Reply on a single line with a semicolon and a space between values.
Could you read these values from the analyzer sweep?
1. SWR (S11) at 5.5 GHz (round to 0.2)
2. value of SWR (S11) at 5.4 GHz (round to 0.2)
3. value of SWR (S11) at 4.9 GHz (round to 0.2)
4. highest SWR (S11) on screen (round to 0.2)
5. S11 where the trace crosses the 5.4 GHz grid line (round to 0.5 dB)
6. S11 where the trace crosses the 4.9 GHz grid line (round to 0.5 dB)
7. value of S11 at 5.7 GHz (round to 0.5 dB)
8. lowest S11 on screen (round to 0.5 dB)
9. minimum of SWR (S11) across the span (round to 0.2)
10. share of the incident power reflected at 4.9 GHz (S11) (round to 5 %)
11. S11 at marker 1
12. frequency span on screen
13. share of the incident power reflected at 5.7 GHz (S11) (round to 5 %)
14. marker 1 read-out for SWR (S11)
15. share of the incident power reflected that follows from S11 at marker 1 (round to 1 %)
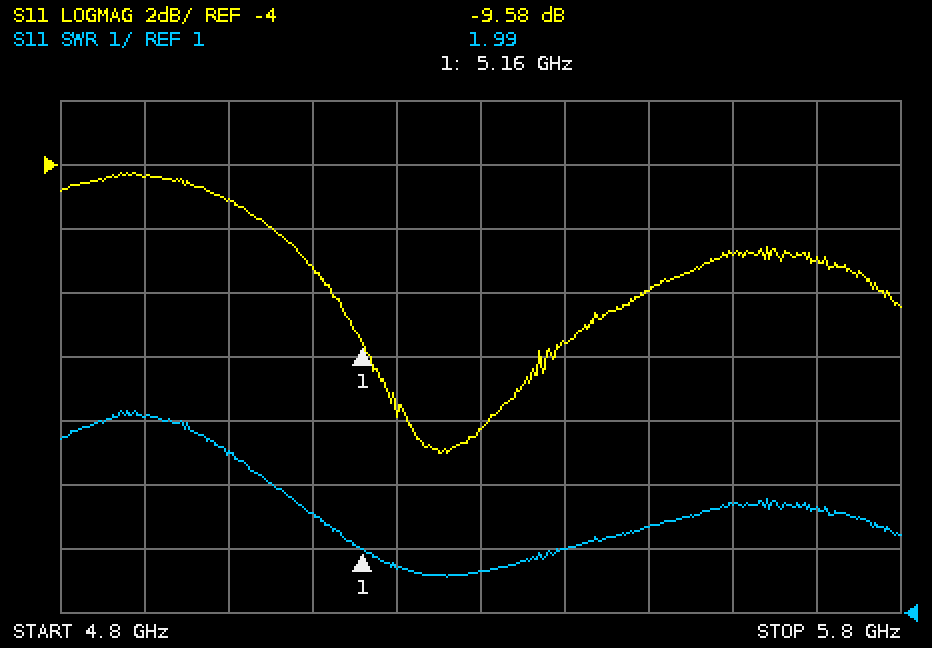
2.4; 2.0; 4.0; 4.2; -9.5 dB; -4.5 dB; -7.0 dB; -13.0 dB; 1.6; 35 %; -9.58 dB; 1 GHz; 20 %; 1.99; 11 %
